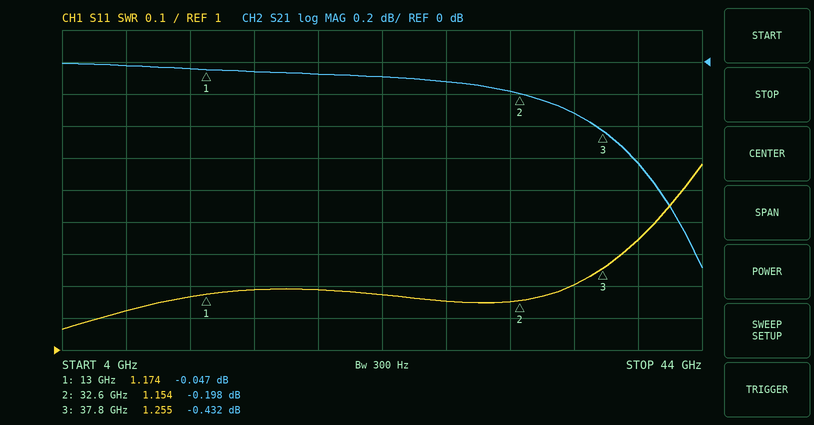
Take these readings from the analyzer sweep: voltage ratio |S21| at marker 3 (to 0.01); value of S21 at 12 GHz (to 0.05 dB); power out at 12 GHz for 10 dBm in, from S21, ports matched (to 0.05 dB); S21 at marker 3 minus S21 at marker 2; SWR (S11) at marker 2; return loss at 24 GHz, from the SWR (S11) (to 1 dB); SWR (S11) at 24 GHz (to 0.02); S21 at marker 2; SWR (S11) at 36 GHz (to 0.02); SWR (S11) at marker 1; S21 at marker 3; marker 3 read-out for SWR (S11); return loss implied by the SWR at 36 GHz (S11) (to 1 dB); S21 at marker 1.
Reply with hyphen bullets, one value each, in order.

- 0.95
- -0.05 dB
- 9.95 dBm
- -0.234 dB
- 1.154
- 22 dB
- 1.18
- -0.198 dB
- 1.20
- 1.174
- -0.432 dB
- 1.255
- 21 dB
- -0.047 dB
